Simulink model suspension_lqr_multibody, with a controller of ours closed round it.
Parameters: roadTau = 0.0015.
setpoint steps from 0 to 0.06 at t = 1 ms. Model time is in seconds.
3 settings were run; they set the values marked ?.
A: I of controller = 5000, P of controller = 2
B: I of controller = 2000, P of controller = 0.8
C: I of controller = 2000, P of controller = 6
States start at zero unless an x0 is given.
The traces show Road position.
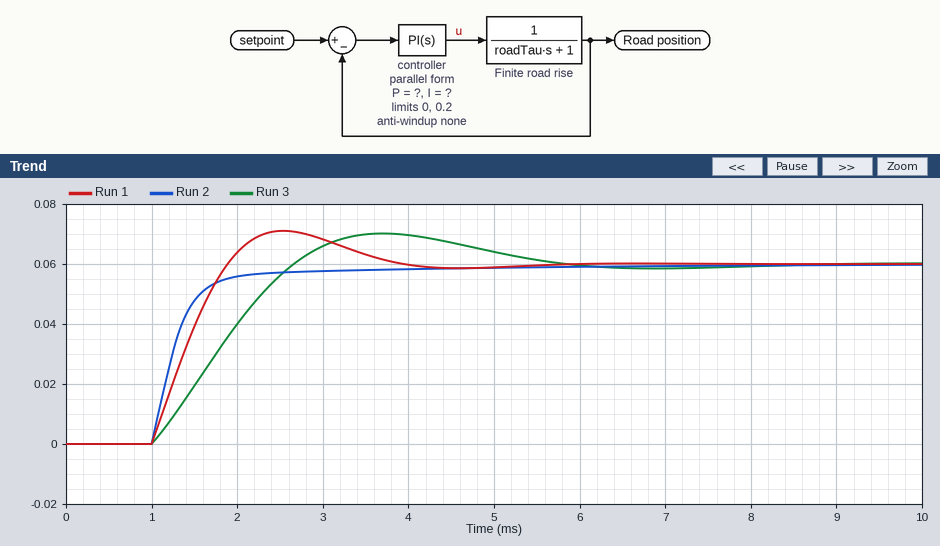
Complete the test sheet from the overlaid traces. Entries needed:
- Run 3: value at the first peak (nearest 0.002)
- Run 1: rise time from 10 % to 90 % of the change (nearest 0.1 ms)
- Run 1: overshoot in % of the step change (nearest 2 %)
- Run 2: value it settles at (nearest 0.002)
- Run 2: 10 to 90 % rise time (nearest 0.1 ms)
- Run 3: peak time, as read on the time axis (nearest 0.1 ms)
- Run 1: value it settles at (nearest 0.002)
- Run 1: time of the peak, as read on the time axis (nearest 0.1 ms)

0.070
0.7 ms
18 %
0.060
0.7 ms
3.7 ms
0.060
2.5 ms
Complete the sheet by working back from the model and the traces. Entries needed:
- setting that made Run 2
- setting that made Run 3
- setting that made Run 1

C
B
A
